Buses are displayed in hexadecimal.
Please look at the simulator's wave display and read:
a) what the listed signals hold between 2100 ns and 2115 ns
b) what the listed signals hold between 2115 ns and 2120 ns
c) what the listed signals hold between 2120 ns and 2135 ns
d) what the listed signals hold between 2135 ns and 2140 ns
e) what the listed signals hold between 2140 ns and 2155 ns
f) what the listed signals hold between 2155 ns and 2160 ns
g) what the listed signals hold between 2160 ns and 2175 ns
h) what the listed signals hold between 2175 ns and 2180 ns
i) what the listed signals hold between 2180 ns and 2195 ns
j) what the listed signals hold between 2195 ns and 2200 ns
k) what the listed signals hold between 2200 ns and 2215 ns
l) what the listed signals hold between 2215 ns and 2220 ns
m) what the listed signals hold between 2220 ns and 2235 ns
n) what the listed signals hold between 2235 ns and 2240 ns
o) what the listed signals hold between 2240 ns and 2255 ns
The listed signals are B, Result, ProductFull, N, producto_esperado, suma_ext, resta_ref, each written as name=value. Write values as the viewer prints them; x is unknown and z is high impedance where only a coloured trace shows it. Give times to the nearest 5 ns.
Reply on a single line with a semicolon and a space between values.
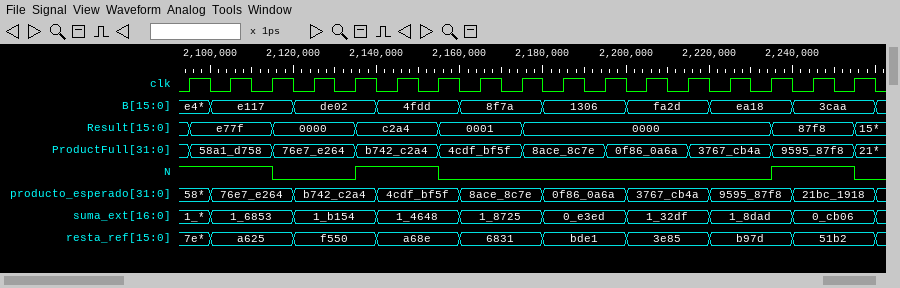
B=e117, Result=e77f, ProductFull=58a1_d758, N=1, producto_esperado=76e7_e264, suma_ext=1_6853, resta_ref=a625; B=e117, Result=0000, ProductFull=76e7_e264, N=0, producto_esperado=76e7_e264, suma_ext=1_6853, resta_ref=a625; B=de02, Result=0000, ProductFull=76e7_e264, N=0, producto_esperado=b742_c2a4, suma_ext=1_b154, resta_ref=f550; B=de02, Result=c2a4, ProductFull=b742_c2a4, N=1, producto_esperado=b742_c2a4, suma_ext=1_b154, resta_ref=f550; B=4fdd, Result=c2a4, ProductFull=b742_c2a4, N=1, producto_esperado=4cdf_bf5f, suma_ext=1_4648, resta_ref=a68e; B=4fdd, Result=0001, ProductFull=4cdf_bf5f, N=0, producto_esperado=4cdf_bf5f, suma_ext=1_4648, resta_ref=a68e; B=8f7a, Result=0001, ProductFull=4cdf_bf5f, N=0, producto_esperado=8ace_8c7e, suma_ext=1_8725, resta_ref=6831; B=8f7a, Result=0000, ProductFull=8ace_8c7e, N=0, producto_esperado=8ace_8c7e, suma_ext=1_8725, resta_ref=6831; B=1306, Result=0000, ProductFull=8ace_8c7e, N=0, producto_esperado=0f86_0a6a, suma_ext=0_e3ed, resta_ref=bde1; B=1306, Result=0000, ProductFull=0f86_0a6a, N=0, producto_esperado=0f86_0a6a, suma_ext=0_e3ed, resta_ref=bde1; B=fa2d, Result=0000, ProductFull=0f86_0a6a, N=0, producto_esperado=3767_cb4a, suma_ext=1_32df, resta_ref=3e85; B=fa2d, Result=0000, ProductFull=3767_cb4a, N=0, producto_esperado=3767_cb4a, suma_ext=1_32df, resta_ref=3e85; B=ea18, Result=0000, ProductFull=3767_cb4a, N=0, producto_esperado=9595_87f8, suma_ext=1_8dad, resta_ref=b97d; B=ea18, Result=87f8, ProductFull=9595_87f8, N=1, producto_esperado=9595_87f8, suma_ext=1_8dad, resta_ref=b97d; B=3caa, Result=87f8, ProductFull=9595_87f8, N=1, producto_esperado=21bc_1918, suma_ext=0_cb06, resta_ref=51b2
